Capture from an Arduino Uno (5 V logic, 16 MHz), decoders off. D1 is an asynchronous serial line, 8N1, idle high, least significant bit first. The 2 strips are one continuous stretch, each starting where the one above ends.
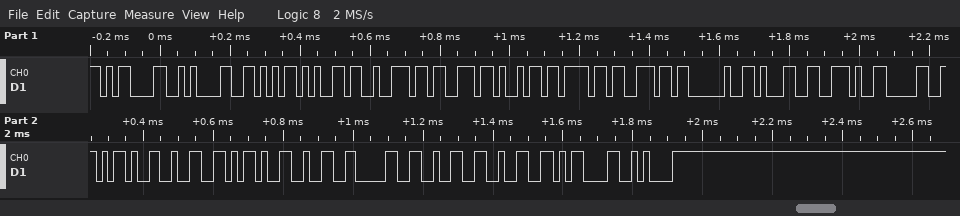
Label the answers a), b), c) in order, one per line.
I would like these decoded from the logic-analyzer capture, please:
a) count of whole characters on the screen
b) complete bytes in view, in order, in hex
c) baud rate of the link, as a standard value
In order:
a) 22
b) 0D 0A 56 65 72 73 69 6F 6E 20 31 2E 30 2D 32 2D 32 30 32 32 0D 0A
c) 57600 baud
